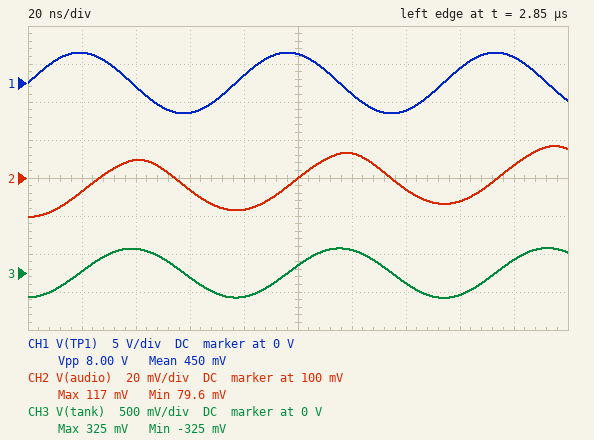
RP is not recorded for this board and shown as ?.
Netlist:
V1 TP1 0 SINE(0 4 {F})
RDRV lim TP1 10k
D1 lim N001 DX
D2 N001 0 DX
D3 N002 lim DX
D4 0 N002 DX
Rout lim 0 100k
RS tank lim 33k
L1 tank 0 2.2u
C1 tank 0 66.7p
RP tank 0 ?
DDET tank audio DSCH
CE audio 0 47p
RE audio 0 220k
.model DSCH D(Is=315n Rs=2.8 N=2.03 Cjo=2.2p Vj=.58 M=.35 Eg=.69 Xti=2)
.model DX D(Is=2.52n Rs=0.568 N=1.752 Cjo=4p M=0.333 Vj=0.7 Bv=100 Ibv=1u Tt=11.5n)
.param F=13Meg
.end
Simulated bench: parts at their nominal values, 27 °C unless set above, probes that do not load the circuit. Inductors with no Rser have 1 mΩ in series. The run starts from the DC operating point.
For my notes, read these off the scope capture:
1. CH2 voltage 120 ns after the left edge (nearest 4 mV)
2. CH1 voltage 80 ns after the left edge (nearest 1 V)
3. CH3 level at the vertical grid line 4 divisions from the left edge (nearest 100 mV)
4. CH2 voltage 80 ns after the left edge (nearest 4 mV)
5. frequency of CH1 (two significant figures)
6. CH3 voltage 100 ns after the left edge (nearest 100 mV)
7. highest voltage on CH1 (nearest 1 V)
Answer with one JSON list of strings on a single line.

["112 mV", "1 V", "-300 mV", "84 mV", "13 MHz", "100 mV", "4 V"]
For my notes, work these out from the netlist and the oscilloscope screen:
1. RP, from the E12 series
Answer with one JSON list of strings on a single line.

["56 kΩ"]
